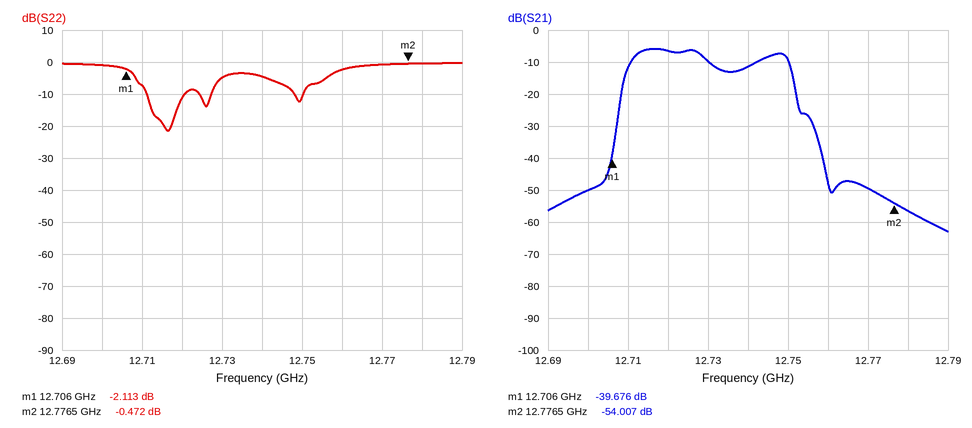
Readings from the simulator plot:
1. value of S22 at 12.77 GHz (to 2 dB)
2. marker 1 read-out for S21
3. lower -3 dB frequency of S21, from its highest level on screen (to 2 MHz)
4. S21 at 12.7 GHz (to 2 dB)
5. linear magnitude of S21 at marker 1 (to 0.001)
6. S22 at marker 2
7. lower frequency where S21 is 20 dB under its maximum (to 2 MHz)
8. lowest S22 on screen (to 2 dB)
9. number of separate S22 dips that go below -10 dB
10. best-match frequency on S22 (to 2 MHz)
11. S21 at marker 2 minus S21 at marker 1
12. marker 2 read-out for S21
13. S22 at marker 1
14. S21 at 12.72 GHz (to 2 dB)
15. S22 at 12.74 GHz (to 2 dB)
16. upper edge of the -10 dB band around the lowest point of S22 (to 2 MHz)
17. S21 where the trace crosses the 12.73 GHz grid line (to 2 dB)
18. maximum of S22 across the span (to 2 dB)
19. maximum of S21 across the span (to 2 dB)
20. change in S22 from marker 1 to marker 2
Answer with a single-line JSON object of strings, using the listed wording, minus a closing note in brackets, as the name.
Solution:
{"value of S22 at 12.77 GHz": "0 dB", "marker 1 read-out for S21": "-39.676 dB", "lower -3 dB frequency of S21, from its highest level on screen": "12.712 GHz", "S21 at 12.7 GHz": "-50 dB", "linear magnitude of S21 at marker 1": "0.010", "S22 at marker 2": "-0.472 dB", "lower frequency where S21 is 20 dB under its maximum": "12.708 GHz", "lowest S22 on screen": "-22 dB", "number of separate S22 dips that go below -10 dB": "3", "best-match frequency on S22": "12.716 GHz", "S21 at marker 2 minus S21 at marker 1": "-14.331 dB", "marker 2 read-out for S21": "-54.007 dB", "S22 at marker 1": "-2.113 dB", "S21 at 12.72 GHz": "-6 dB", "S22 at 12.74 GHz": "-4 dB", "upper edge of the -10 dB band around the lowest point of S22": "12.720 GHz", "S21 where the trace crosses the 12.73 GHz grid line": "-10 dB", "maximum of S22 across the span": "0 dB", "maximum of S21 across the span": "-6 dB", "change in S22 from marker 1 to marker 2": "1.641 dB"}
